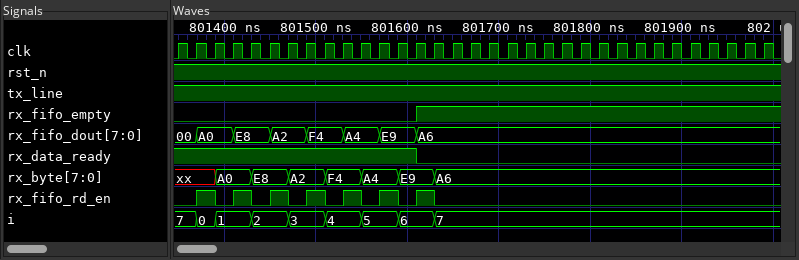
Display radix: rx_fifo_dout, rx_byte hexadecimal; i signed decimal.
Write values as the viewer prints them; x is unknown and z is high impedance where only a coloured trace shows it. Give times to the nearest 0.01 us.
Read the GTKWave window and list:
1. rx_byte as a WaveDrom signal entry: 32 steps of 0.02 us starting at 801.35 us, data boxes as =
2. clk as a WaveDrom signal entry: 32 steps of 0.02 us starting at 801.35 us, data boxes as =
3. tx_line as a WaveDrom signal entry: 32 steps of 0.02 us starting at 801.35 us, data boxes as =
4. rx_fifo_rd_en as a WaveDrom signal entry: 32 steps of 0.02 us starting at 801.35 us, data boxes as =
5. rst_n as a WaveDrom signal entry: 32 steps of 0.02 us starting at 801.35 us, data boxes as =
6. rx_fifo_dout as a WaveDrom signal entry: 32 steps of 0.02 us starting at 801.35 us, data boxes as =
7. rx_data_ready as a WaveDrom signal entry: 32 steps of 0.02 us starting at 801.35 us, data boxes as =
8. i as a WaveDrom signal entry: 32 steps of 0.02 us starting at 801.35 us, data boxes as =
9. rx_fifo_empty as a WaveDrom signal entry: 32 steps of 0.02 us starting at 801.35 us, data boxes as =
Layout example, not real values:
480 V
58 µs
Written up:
{name: 'rx_byte', wave: 'x.=.=.=.=.=.=.=.................', data: 'A0 E8 A2 F4 A4 E9 A6'}
{name: 'clk', wave: 'p...............................'}
{name: 'tx_line', wave: '1...............................'}
{name: 'rx_fifo_rd_en', wave: '010101010101010.................'}
{name: 'rst_n', wave: '1...............................'}
{name: 'rx_fifo_dout', wave: '==.=.=.=.=.=.=..................', data: '00 A0 E8 A2 F4 A4 E9 A6'}
{name: 'rx_data_ready', wave: '1............0..................'}
{name: 'i', wave: '===.=.=.=.=.=.=.................', data: '7 0 1 2 3 4 5 6 7'}
{name: 'rx_fifo_empty', wave: '0............1..................'}
